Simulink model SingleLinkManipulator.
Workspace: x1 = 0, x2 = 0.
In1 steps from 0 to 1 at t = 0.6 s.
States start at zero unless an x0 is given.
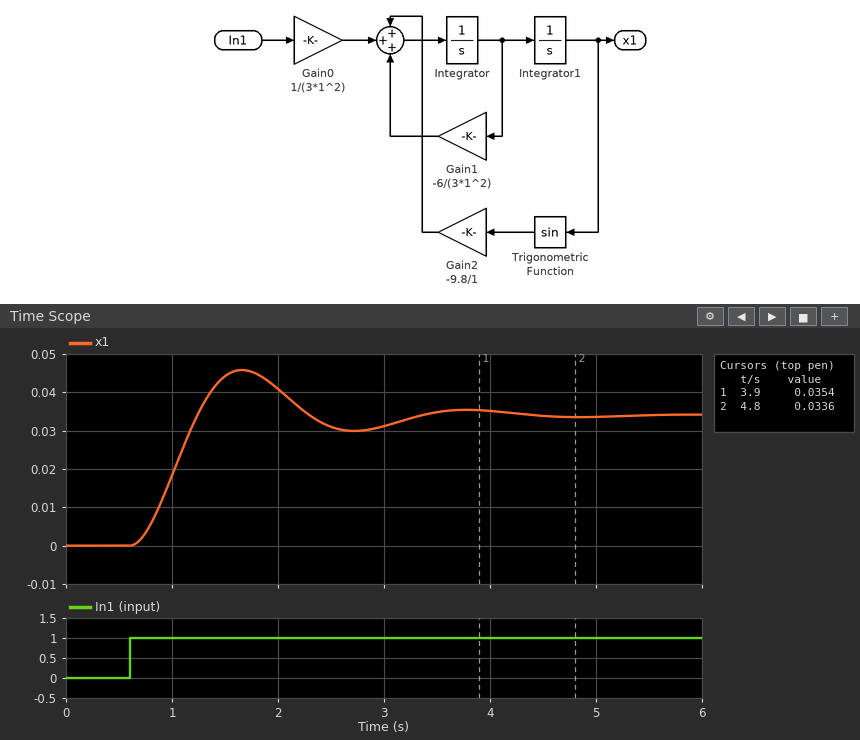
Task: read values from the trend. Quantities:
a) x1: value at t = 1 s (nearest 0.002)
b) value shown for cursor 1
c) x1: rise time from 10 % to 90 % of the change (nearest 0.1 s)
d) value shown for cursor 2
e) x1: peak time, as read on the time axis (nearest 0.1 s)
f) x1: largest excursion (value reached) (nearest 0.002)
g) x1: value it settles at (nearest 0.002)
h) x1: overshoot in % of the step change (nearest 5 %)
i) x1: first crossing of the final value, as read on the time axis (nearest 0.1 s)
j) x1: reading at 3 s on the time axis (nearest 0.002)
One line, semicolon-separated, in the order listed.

0.018; 0.0354; 0.4 s; 0.0336; 1.7 s; 0.046; 0.034; 35 %; 1.2 s; 0.032
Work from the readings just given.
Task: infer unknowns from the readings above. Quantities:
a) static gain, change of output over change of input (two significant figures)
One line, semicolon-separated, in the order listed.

0.034
